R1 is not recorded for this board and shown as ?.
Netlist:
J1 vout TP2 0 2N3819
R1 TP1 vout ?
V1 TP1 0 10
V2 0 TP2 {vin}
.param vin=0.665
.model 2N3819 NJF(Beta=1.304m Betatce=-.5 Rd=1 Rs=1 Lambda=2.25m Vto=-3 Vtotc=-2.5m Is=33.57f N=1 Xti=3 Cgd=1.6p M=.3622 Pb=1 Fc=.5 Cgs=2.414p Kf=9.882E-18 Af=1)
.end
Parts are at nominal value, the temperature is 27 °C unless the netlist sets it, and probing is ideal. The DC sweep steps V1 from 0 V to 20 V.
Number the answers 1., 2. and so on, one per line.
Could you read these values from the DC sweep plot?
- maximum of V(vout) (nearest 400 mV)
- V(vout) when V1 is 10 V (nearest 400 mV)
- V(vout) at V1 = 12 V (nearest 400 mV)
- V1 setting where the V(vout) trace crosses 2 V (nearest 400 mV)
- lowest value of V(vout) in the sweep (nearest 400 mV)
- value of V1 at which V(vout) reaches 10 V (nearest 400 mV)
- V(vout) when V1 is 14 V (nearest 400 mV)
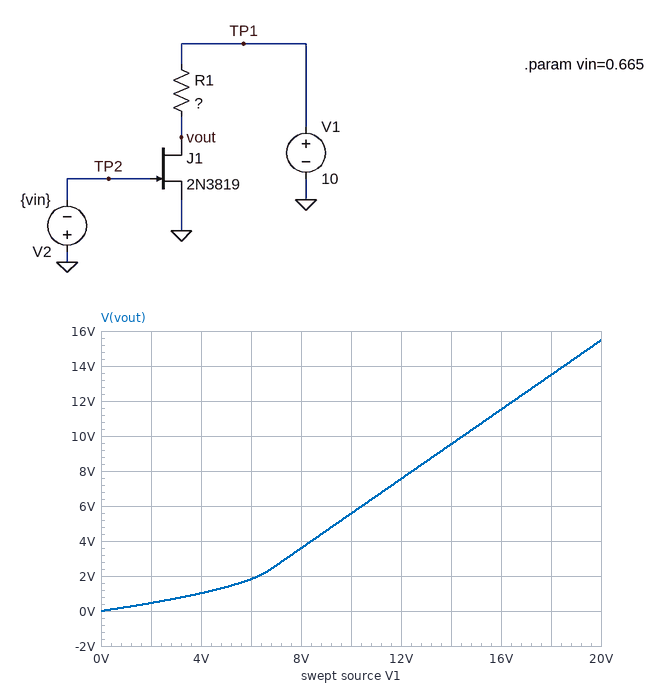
1. 15.6 V
2. 5.6 V
3. 7.6 V
4. 6.4 V
5. 0 V
6. 14.4 V
7. 9.6 V
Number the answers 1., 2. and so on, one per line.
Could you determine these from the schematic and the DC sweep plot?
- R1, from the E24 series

1. 620 Ω
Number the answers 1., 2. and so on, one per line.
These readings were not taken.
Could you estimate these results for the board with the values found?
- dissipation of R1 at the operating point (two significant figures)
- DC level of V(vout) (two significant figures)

1. 32 mW
2. 5.6 V
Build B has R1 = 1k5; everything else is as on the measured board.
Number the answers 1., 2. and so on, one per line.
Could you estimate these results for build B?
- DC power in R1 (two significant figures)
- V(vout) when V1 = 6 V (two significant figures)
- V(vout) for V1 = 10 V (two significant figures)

1. 50 mW
2. 690 mV
3. 1.3 V
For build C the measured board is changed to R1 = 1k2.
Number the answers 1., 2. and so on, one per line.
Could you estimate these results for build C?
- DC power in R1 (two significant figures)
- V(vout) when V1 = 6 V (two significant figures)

1. 55 mW
2. 870 mV
